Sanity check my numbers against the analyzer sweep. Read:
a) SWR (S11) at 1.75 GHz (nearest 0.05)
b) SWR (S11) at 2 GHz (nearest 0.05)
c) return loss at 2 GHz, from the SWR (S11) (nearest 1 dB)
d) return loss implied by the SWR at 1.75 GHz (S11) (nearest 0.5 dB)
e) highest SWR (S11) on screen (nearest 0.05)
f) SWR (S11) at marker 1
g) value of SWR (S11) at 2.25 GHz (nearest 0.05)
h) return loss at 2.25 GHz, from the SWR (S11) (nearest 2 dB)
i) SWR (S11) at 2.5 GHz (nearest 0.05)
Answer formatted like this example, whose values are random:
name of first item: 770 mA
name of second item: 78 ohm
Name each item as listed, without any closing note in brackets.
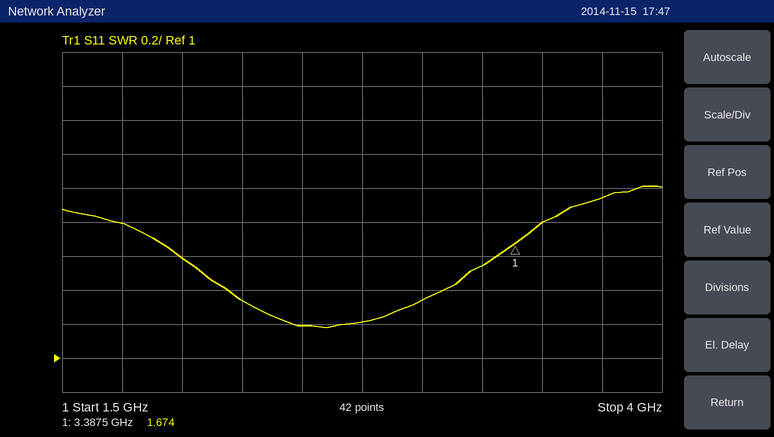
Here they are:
SWR (S11) at 1.75 GHz: 1.80
SWR (S11) at 2 GHz: 1.60
return loss at 2 GHz, from the SWR (S11): 13 dB
return loss implied by the SWR at 1.75 GHz (S11): 11.0 dB
highest SWR (S11) on screen: 2.00
SWR (S11) at marker 1: 1.674
value of SWR (S11) at 2.25 GHz: 1.35
return loss at 2.25 GHz, from the SWR (S11): 16 dB
SWR (S11) at 2.5 GHz: 1.20
